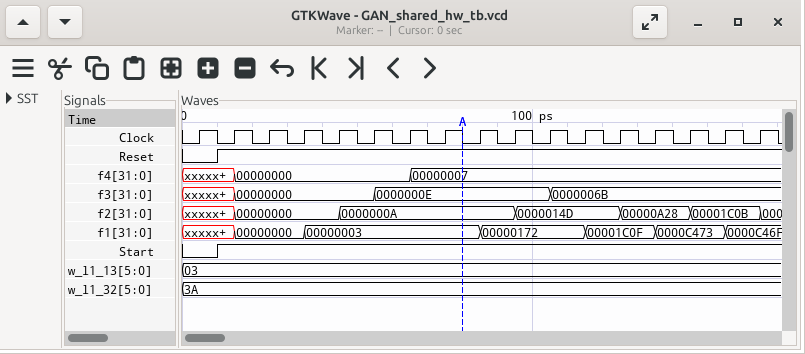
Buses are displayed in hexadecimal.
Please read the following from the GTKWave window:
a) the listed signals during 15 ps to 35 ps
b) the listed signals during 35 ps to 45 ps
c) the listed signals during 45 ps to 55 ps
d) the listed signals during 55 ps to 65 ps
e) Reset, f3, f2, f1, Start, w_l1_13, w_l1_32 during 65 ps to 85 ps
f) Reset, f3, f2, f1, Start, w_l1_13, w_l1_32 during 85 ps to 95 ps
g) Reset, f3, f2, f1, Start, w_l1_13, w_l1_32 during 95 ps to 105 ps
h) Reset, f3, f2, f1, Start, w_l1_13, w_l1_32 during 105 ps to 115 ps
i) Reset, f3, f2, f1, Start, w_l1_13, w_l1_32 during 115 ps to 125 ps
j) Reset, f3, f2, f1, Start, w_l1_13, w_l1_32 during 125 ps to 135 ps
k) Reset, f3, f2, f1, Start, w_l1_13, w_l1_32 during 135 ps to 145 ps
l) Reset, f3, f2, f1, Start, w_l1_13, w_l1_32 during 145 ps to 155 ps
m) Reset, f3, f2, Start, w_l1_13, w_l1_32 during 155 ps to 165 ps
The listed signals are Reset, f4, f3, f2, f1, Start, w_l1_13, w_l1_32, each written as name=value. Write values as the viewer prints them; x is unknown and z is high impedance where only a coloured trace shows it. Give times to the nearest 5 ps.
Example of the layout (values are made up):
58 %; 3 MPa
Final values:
Reset=1, f4=00000000, f3=00000000, f2=00000000, f1=00000000, Start=1, w_l1_13=03, w_l1_32=3A; Reset=1, f4=00000000, f3=00000000, f2=00000000, f1=00000003, Start=1, w_l1_13=03, w_l1_32=3A; Reset=1, f4=00000000, f3=00000000, f2=0000000A, f1=00000003, Start=1, w_l1_13=03, w_l1_32=3A; Reset=1, f4=00000000, f3=0000000E, f2=0000000A, f1=00000003, Start=1, w_l1_13=03, w_l1_32=3A; Reset=1, f3=0000000E, f2=0000000A, f1=00000003, Start=1, w_l1_13=03, w_l1_32=3A; Reset=1, f3=0000000E, f2=0000000A, f1=00000172, Start=1, w_l1_13=03, w_l1_32=3A; Reset=1, f3=0000000E, f2=0000014D, f1=00000172, Start=1, w_l1_13=03, w_l1_32=3A; Reset=1, f3=0000006B, f2=0000014D, f1=00000172, Start=1, w_l1_13=03, w_l1_32=3A; Reset=1, f3=0000006B, f2=0000014D, f1=00001C0F, Start=1, w_l1_13=03, w_l1_32=3A; Reset=1, f3=0000006B, f2=00000A28, f1=00001C0F, Start=1, w_l1_13=03, w_l1_32=3A; Reset=1, f3=0000006B, f2=00000A28, f1=0000C473, Start=1, w_l1_13=03, w_l1_32=3A; Reset=1, f3=0000006B, f2=00001C0B, f1=0000C473, Start=1, w_l1_13=03, w_l1_32=3A; Reset=1, f3=0000006B, f2=00001C0B, Start=1, w_l1_13=03, w_l1_32=3A
